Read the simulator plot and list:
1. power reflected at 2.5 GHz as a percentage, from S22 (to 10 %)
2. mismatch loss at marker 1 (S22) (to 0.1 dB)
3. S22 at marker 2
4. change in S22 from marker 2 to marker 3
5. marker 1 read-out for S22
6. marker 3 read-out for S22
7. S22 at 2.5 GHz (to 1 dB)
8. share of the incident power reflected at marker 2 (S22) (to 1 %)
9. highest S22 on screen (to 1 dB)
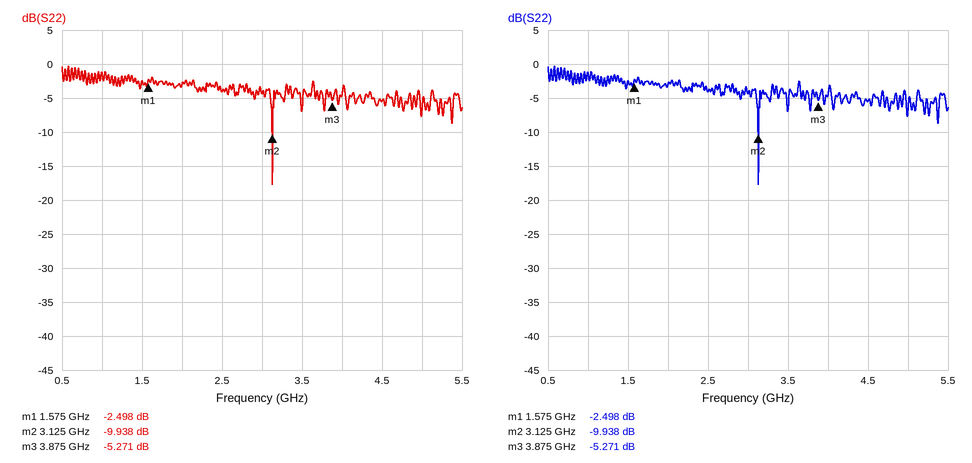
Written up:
40 %
3.6 dB
-9.938 dB
4.667 dB
-2.498 dB
-5.271 dB
-4 dB
10 %
0 dB
